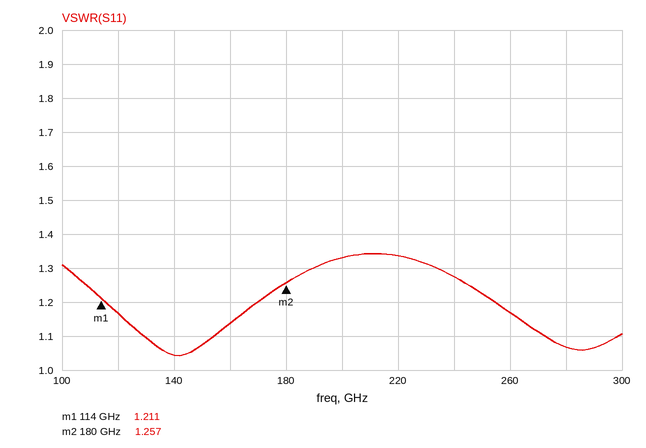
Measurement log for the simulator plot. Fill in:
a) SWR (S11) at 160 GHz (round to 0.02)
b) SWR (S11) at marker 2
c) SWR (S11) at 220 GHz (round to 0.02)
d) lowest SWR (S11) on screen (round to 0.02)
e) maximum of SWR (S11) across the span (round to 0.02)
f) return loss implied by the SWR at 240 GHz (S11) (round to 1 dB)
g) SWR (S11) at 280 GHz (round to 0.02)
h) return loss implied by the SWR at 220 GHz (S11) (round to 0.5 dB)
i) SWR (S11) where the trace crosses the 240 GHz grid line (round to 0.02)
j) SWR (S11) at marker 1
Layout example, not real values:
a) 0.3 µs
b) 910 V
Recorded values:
a) 1.14
b) 1.257
c) 1.34
d) 1.04
e) 1.34
f) 18 dB
g) 1.06
h) 17.0 dB
i) 1.28
j) 1.211
